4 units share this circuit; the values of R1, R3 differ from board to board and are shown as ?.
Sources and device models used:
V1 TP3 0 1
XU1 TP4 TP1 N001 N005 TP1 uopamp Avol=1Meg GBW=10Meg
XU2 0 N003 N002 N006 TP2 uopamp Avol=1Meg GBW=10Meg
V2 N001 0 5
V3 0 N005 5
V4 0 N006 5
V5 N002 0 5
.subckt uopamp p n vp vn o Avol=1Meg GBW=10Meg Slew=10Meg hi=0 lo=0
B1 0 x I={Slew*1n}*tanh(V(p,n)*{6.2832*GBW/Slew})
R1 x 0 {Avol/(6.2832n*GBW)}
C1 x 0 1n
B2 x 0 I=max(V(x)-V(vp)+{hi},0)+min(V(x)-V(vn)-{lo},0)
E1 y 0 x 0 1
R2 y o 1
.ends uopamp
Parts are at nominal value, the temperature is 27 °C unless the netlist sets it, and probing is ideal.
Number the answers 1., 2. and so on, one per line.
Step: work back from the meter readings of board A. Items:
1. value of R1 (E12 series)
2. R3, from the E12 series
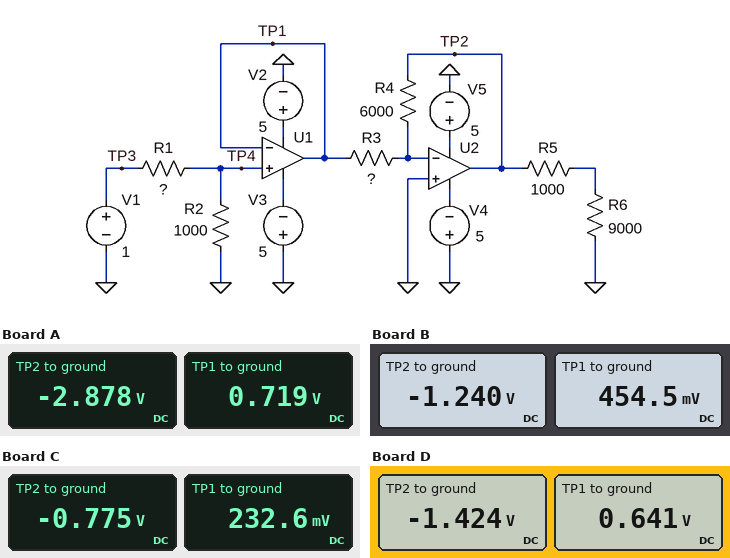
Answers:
1. 390 Ω
2. 1.5 kΩ
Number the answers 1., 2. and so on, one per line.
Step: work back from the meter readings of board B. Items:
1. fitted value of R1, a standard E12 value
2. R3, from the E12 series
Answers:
1. 1.2 kΩ
2. 2.2 kΩ
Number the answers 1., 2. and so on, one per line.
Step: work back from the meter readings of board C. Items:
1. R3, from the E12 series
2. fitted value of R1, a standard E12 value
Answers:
1. 1.8 kΩ
2. 3.3 kΩ
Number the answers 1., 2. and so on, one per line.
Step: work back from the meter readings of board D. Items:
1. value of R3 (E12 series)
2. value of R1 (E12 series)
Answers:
1. 2.7 kΩ
2. 560 Ω
